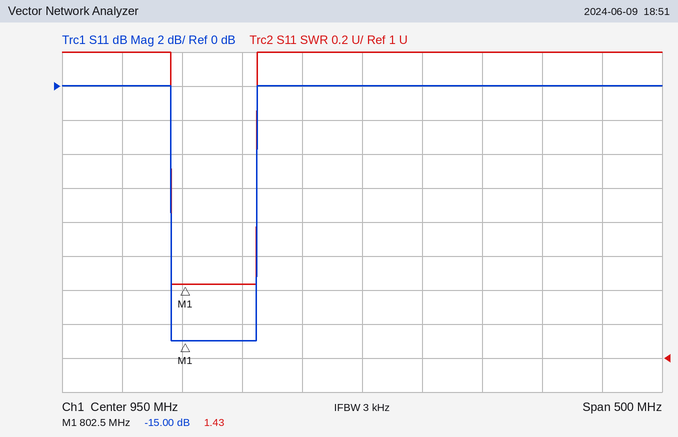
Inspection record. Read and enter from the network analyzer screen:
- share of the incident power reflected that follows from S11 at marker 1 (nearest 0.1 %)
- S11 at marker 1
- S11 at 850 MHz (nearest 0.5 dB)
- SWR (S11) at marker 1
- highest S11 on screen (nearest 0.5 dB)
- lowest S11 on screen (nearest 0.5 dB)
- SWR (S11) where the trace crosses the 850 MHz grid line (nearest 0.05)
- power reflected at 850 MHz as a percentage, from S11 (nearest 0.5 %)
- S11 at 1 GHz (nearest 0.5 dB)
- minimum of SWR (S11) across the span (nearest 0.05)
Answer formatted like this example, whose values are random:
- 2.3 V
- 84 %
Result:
- 3.2 %
- -15.00 dB
- -15.0 dB
- 1.43
- 0.0 dB
- -15.0 dB
- 1.45
- 3.0 %
- 0.0 dB
- 1.45
